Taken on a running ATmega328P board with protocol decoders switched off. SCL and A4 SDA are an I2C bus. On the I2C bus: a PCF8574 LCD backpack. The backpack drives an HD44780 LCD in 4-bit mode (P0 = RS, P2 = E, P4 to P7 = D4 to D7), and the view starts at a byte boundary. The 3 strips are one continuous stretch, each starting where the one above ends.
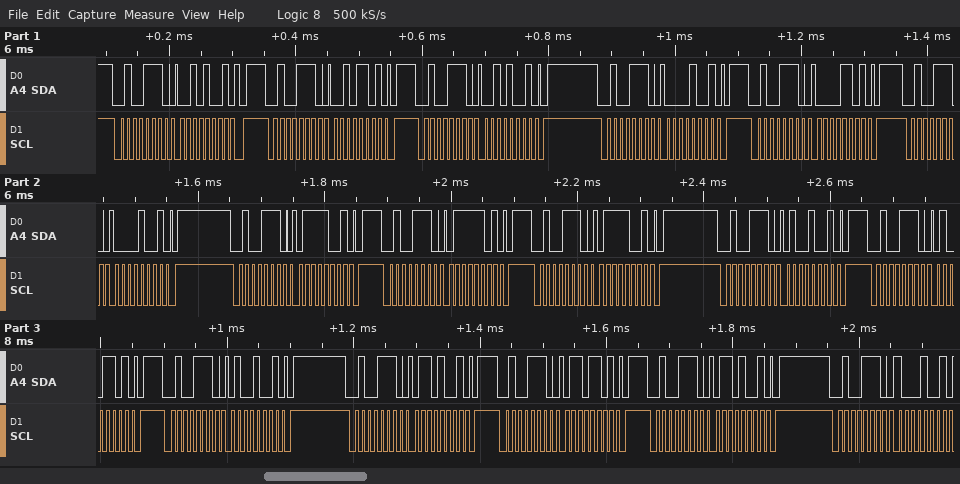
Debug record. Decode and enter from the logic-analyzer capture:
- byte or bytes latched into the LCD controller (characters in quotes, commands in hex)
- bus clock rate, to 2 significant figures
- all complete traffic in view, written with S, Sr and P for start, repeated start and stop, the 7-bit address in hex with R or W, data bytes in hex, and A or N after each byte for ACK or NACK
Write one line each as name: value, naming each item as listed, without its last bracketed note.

byte or bytes latched into the LCD controller: ' ' 't'
bus clock rate, to 2 significant figures: 100 kHz
all complete traffic in view, written with S, Sr and P for start, repeated start and stop, the 7-bit address in hex with R or W, data bytes in hex, and A or N after each byte for ACK or NACK: S 27W A 29 A P S 27W A 2D A P S 27W A 29 A P S 27W A 09 A P S 27W A 0D A P S 27W A 09 A P S 27W A 79 A P S 27W A 7D A P S 27W A 79 A P S 27W A 49 A P S 27W A 4D A P S 27W A 49 A P S 27W A 69 A P S 27W A 6D A P S 27W A 69 A P S 27W A 89 A
